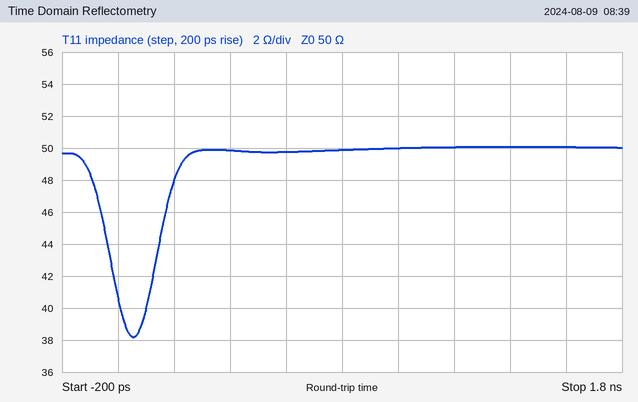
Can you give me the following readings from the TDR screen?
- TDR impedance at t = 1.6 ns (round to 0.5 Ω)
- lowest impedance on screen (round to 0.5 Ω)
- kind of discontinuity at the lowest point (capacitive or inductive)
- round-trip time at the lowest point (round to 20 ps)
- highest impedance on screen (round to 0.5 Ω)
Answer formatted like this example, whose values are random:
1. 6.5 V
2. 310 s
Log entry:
1. 50.0 Ω
2. 38.0 Ω
3. capacitive
4. 60 ps
5. 50.0 Ω
